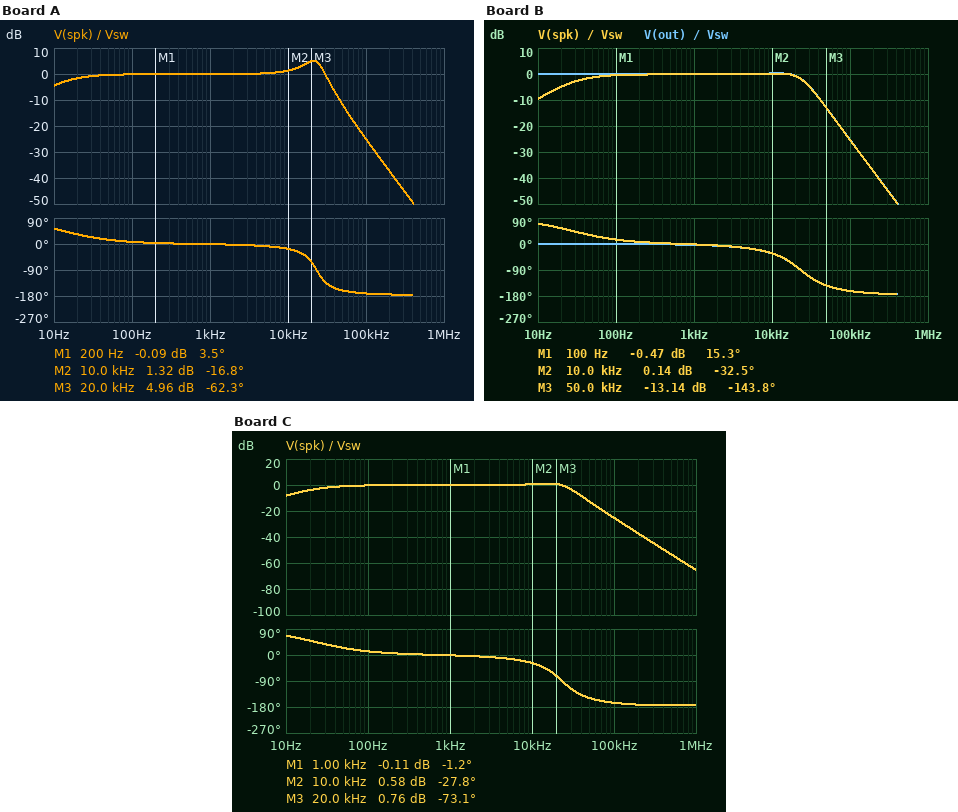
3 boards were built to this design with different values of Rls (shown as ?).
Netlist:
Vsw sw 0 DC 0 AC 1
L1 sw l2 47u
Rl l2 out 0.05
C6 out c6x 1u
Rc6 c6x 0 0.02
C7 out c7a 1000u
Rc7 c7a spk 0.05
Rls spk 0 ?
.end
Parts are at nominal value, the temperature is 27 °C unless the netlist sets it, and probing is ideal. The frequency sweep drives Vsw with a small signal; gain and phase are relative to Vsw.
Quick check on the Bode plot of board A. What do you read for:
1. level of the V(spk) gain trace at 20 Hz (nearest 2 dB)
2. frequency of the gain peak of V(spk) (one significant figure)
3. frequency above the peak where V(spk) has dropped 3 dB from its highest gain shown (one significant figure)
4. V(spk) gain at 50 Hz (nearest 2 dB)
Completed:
-2 dB
20 kHz
30 kHz
0 dB
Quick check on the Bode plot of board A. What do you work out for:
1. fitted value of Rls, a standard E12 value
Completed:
12 Ω
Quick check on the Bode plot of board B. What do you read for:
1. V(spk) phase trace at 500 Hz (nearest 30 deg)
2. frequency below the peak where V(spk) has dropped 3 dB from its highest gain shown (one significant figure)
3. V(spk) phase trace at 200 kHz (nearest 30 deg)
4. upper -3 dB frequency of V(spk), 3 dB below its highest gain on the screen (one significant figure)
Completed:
0 deg
30 Hz
-180 deg
30 kHz
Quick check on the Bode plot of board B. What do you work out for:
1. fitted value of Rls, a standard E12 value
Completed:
5.6 Ω
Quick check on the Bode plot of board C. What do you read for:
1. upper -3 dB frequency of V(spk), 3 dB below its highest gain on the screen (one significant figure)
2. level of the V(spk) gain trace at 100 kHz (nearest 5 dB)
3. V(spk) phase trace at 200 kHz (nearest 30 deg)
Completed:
30 kHz
-25 dB
-180 deg
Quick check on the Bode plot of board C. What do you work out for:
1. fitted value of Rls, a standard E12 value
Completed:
6.8 Ω
